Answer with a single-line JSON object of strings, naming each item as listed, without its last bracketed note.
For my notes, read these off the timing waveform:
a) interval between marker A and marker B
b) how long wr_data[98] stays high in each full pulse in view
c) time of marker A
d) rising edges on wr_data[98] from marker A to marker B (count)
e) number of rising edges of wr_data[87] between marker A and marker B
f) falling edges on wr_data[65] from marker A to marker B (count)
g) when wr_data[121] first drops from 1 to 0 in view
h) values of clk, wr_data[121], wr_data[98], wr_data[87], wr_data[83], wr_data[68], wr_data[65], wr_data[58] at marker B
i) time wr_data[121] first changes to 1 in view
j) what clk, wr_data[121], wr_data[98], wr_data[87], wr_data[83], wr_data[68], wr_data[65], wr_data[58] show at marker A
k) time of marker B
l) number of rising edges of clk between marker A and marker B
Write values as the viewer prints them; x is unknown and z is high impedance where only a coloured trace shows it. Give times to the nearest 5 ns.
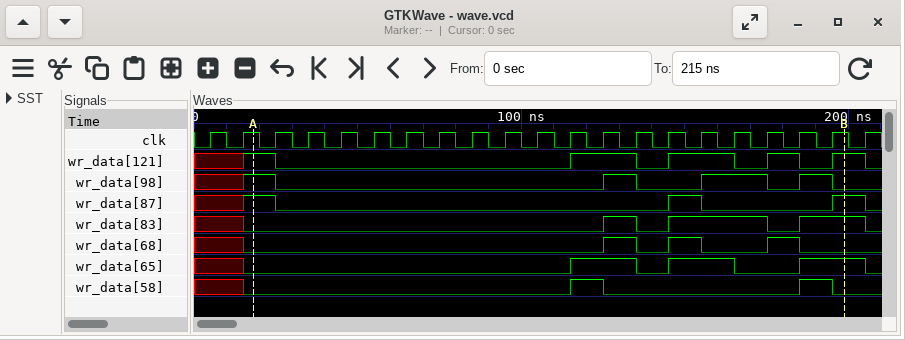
{"interval between marker A and marker B": "180 ns", "how long wr_data[98] stays high in each full pulse in view": "10 ns, 20 ns, 10 ns", "time of marker A": "20 ns", "rising edges on wr_data[98] from marker A to marker B": "3", "number of rising edges of wr_data[87] between marker A and marker B": "2", "falling edges on wr_data[65] from marker A to marker B": "2", "when wr_data[121] first drops from 1 to 0 in view": "25 ns", "values of clk, wr_data[121], wr_data[98], wr_data[87], wr_data[83], wr_data[68], wr_data[65], wr_data[58] at marker B": "clk=1, wr_data[121]=1, wr_data[98]=0, wr_data[87]=1, wr_data[83]=1, wr_data[68]=0, wr_data[65]=1, wr_data[58]=0", "time wr_data[121] first changes to 1 in view": "15 ns", "what clk, wr_data[121], wr_data[98], wr_data[87], wr_data[83], wr_data[68], wr_data[65], wr_data[58] show at marker A": "clk=1, wr_data[121]=1, wr_data[98]=1, wr_data[87]=1, wr_data[83]=0, wr_data[68]=0, wr_data[65]=0, wr_data[58]=0", "time of marker B": "200 ns", "number of rising edges of clk between marker A and marker B": "18"}
